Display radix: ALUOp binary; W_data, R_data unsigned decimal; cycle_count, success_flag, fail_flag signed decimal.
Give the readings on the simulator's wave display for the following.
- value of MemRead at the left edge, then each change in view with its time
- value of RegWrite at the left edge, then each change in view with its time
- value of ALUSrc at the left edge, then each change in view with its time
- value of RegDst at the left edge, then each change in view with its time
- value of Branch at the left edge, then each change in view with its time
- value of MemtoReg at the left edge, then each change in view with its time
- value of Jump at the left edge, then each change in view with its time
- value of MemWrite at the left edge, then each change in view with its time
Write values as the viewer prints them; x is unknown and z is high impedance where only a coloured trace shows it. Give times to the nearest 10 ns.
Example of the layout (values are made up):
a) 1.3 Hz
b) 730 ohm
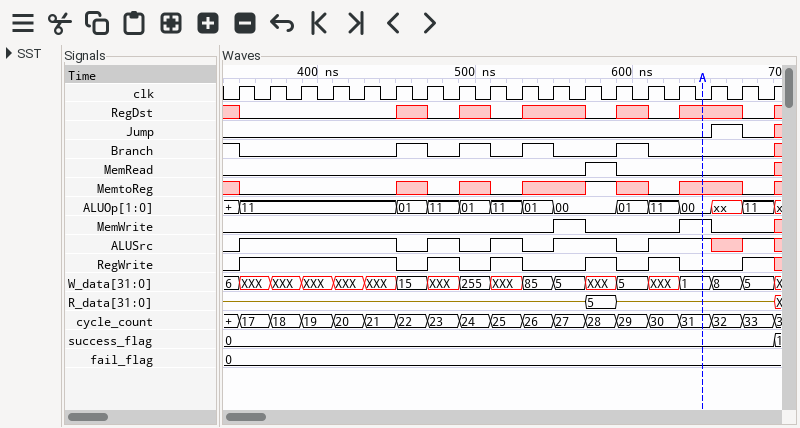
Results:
a) 0, 1 at 570 ns, 0 at 590 ns, x at 690 ns
b) 0, 1 at 350 ns, 0 at 450 ns, 1 at 470 ns, 0 at 490 ns, 1 at 510 ns, 0 at 530 ns, 1 at 570 ns, 0 at 590 ns, 1 at 610 ns, 0 at 630 ns, 1 at 670 ns, x at 690 ns
c) 0, 1 at 350 ns, 0 at 450 ns, 1 at 470 ns, 0 at 490 ns, 1 at 510 ns, 0 at 530 ns, 1 at 550 ns, 0 at 590 ns, 1 at 610 ns, x at 650 ns, 1 at 670 ns, x at 690 ns
d) x, 0 at 350 ns, x at 450 ns, 0 at 470 ns, x at 490 ns, 0 at 510 ns, x at 530 ns, 0 at 570 ns, x at 590 ns, 0 at 610 ns, x at 630 ns, 0 at 670 ns, x at 690 ns
e) 1, 0 at 350 ns, 1 at 450 ns, 0 at 470 ns, 1 at 490 ns, 0 at 510 ns, 1 at 530 ns, 0 at 550 ns, 1 at 590 ns, 0 at 610 ns, x at 690 ns
f) x, 0 at 350 ns, x at 450 ns, 0 at 470 ns, x at 490 ns, 0 at 510 ns, x at 530 ns, 1 at 570 ns, x at 590 ns, 0 at 610 ns, x at 630 ns, 0 at 670 ns, x at 690 ns
g) 0, 1 at 650 ns, 0 at 670 ns, x at 690 ns
h) 0, 1 at 550 ns, 0 at 570 ns, 1 at 630 ns, 0 at 650 ns, x at 690 ns
